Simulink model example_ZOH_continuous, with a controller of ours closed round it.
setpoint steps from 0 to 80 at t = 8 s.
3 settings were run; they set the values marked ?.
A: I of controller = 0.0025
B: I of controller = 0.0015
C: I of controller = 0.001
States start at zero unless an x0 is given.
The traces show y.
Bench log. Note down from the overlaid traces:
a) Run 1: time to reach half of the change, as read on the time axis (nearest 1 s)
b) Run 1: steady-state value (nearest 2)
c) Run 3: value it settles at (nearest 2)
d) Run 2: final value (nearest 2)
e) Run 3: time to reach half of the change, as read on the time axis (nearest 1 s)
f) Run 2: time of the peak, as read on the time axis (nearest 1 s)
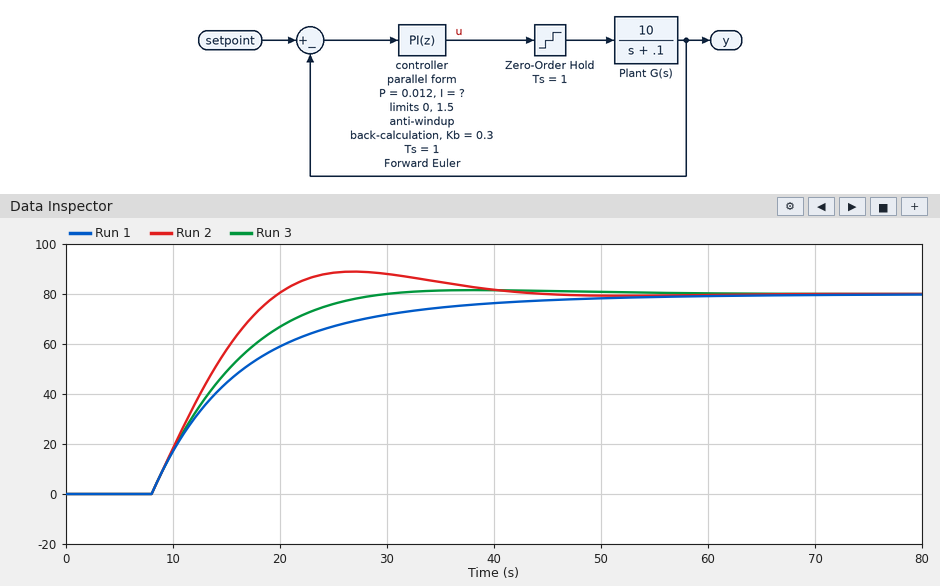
14 s
80
80
80
13 s
27 s
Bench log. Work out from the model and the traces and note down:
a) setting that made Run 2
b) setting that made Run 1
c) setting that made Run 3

A
C
B
